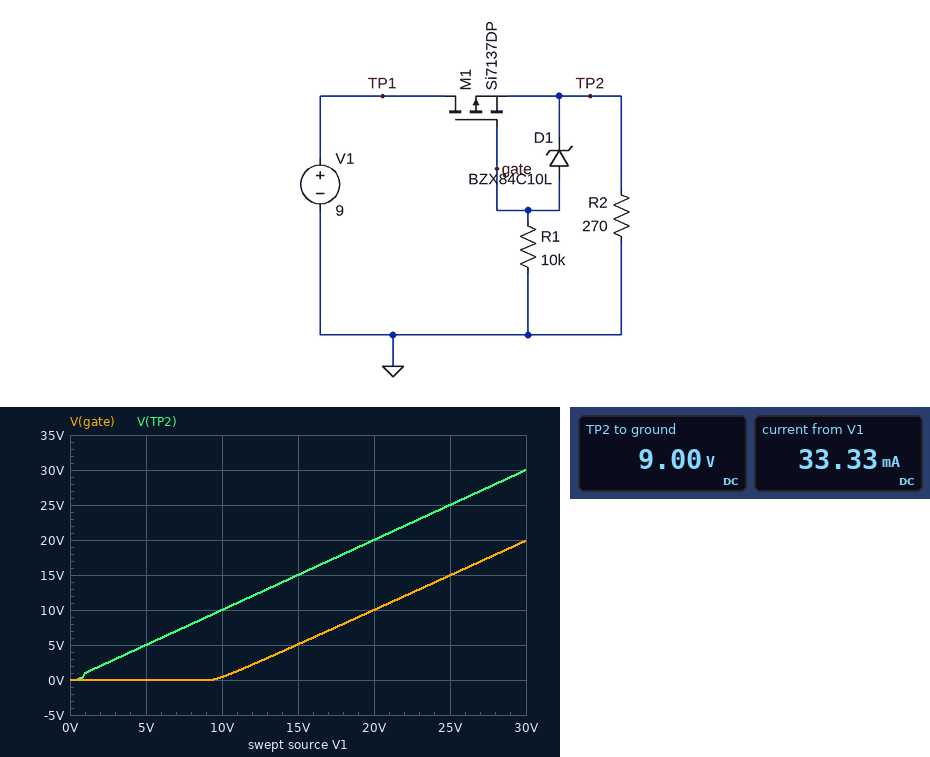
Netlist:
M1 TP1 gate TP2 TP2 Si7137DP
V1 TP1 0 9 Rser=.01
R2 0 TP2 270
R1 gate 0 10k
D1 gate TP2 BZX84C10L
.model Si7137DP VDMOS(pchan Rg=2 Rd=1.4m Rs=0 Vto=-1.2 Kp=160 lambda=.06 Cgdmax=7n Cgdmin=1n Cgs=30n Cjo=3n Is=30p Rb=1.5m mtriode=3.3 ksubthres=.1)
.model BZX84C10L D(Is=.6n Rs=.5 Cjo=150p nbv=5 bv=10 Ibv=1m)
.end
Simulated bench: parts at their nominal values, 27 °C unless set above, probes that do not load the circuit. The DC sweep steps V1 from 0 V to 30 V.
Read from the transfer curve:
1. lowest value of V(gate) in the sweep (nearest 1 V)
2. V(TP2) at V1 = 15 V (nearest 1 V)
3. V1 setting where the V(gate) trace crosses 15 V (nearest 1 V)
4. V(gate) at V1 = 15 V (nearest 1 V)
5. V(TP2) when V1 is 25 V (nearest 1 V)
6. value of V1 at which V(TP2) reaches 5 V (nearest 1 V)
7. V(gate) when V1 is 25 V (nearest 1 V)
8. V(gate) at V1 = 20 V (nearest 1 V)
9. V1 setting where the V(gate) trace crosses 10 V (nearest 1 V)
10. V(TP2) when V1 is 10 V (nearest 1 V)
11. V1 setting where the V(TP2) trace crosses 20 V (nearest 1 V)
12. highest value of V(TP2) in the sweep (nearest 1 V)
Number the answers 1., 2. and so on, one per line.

1. 0 V
2. 15 V
3. 25 V
4. 5 V
5. 25 V
6. 5 V
7. 15 V
8. 10 V
9. 20 V
10. 10 V
11. 20 V
12. 30 V
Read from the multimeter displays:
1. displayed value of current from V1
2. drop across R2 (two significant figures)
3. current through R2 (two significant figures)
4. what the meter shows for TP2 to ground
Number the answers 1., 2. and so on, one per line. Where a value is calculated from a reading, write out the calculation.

1. 33.33 mA
2. 9 V = 9.0 V
3. (9 V) / 270 Ω = 33 mA
4. 9.00 V
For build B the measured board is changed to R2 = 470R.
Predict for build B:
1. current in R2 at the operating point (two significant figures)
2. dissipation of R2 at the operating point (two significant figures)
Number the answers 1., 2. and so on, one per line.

1. 19 mA
2. 170 mW
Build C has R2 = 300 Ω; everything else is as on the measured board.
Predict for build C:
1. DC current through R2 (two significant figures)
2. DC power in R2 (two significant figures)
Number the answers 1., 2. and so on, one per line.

1. 30 mA
2. 270 mW
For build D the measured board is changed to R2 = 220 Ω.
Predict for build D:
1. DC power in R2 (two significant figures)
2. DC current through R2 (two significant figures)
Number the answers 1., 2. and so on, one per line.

1. 370 mW
2. 41 mA
